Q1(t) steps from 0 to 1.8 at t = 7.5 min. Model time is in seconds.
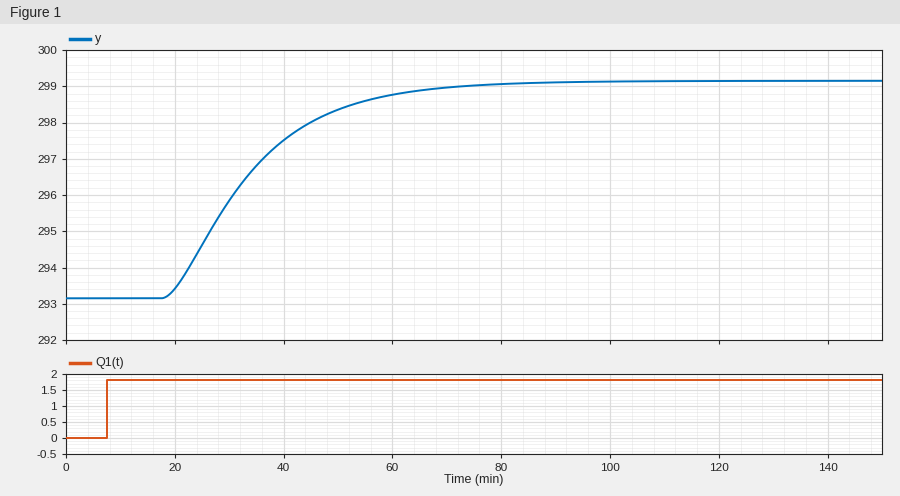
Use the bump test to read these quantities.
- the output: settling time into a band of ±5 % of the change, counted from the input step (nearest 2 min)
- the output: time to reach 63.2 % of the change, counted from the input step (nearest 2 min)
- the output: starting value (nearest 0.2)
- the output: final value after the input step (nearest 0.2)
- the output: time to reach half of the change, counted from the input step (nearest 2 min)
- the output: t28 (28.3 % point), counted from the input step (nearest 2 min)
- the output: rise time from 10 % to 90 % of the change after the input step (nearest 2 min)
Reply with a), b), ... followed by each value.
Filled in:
a) 56 min
b) 28 min
c) 293.2
d) 299.2
e) 24 min
f) 18 min
g) 32 min
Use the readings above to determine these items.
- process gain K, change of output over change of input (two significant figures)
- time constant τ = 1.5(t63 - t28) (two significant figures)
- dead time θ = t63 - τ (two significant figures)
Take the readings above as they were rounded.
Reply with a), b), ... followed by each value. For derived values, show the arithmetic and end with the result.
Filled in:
a) (299.2 - 293.2) / 1.8 = 3.3
b) 1.5 × (28 - 18) = 15 min
c) 28 - 15 = 13 min
